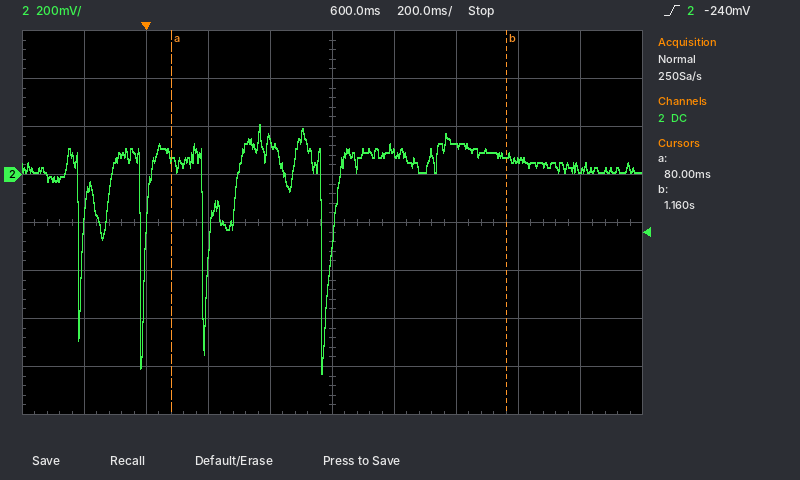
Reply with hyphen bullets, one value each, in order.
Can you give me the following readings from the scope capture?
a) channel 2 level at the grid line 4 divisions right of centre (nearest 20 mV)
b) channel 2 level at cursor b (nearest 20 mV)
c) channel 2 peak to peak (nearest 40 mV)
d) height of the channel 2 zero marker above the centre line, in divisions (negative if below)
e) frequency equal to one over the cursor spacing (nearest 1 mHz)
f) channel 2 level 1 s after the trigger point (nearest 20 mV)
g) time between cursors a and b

- 20 mV
- 80 mV
- 1.04 V
- +1.0 div
- 926 mHz
- 120 mV
- 1.08 s
